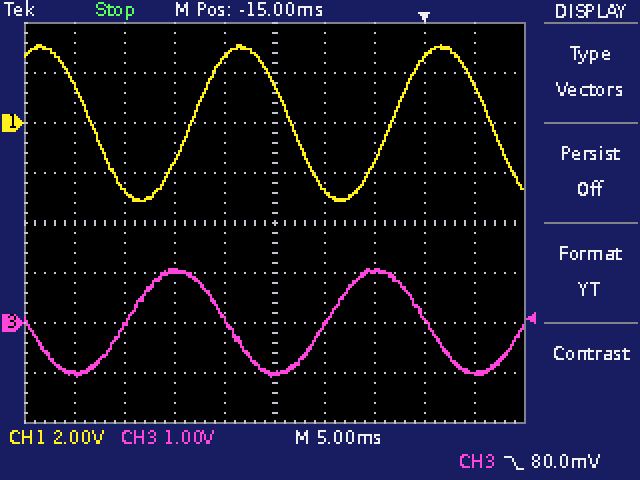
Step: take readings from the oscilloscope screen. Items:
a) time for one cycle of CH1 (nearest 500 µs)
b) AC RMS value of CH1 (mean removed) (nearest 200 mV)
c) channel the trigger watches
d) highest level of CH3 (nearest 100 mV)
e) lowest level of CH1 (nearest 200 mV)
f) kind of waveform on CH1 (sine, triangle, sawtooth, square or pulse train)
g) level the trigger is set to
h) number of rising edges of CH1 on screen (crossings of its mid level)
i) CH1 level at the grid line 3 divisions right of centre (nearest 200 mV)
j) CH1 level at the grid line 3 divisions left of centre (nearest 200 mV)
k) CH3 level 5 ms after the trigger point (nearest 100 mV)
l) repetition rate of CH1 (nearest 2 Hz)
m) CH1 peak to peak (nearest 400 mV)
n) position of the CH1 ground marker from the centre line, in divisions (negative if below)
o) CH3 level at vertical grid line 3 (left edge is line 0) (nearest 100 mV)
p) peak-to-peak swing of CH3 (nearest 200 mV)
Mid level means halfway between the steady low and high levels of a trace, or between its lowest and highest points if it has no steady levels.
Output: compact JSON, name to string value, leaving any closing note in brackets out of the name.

{"time for one cycle of CH1": "20.0 ms", "AC RMS value of CH1 (mean removed)": "2.2 V", "channel the trigger watches": "CH3", "highest level of CH3": "1.1 V", "lowest level of CH1": "-3.2 V", "kind of waveform on CH1": "sine", "level the trigger is set to": "80.0 mV", "number of rising edges of CH1 on screen": "2", "CH1 level at the grid line 3 divisions right of centre": "2.6 V", "CH1 level at the grid line 3 divisions left of centre": "-2.6 V", "CH3 level 5 ms after the trigger point": "-1.0 V", "repetition rate of CH1": "50 Hz", "CH1 peak to peak": "6.4 V", "position of the CH1 ground marker from the centre line, in divisions": "+2.0 div", "CH3 level at vertical grid line 3 (left edge is line 0)": "1.0 V", "peak-to-peak swing of CH3": "2.2 V"}
